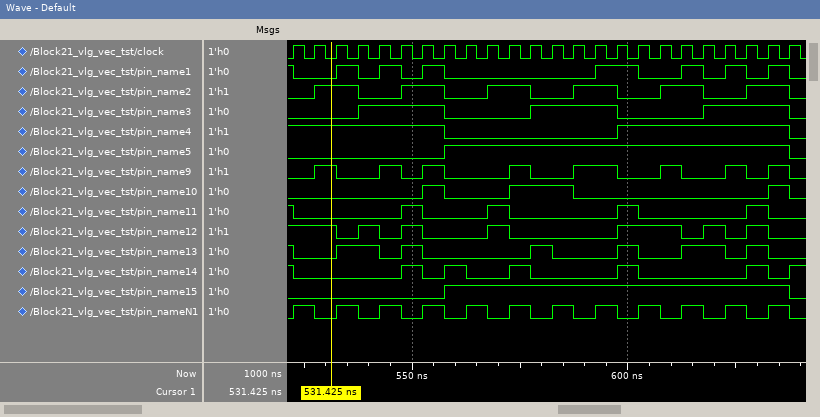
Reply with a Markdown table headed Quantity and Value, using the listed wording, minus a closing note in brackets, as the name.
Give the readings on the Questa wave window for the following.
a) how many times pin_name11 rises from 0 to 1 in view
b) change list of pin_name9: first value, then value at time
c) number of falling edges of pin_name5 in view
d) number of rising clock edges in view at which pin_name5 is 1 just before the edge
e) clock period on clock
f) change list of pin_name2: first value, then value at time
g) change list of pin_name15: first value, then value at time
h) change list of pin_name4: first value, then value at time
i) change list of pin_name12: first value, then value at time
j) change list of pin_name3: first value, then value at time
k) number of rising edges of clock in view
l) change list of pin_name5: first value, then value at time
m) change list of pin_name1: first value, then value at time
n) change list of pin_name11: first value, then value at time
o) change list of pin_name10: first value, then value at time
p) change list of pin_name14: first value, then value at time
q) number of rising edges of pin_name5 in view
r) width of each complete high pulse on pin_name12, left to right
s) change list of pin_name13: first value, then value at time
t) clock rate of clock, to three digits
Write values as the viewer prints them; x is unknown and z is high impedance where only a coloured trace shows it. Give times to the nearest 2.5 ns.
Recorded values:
| Quantity | Value |
|---|---|
| how many times pin_name11 rises from 0 to 1 in view | 4 |
| change list of pin_name9: first value, then value at time | 0, 1 at 527.5 ns, 0 at 532.5 ns, 1 at 542.5 ns, 0 at 547.5 ns, 1 at 552.5 ns, 0 at 557.5 ns, 1 at 572.5 ns, 0 at 577.5 ns, 1 at 587.5 ns, 0 at 597.5 ns, 1 at 607.5 ns, 0 at 612.5 ns, 1 at 622.5 ns, 0 at 627.5 ns, 1 at 632.5 ns, 0 at 637.5 ns |
| number of falling edges of pin_name5 in view | 1 |
| number of rising clock edges in view at which pin_name5 is 1 just before the edge | 16 |
| clock period on clock | 5 ns |
| change list of pin_name2: first value, then value at time | 0, 1 at 527.5 ns, 0 at 537.5 ns, 1 at 547.5 ns, 0 at 557.5 ns, 1 at 567.5 ns, 0 at 577.5 ns, 1 at 587.5 ns, 0 at 597.5 ns, 1 at 607.5 ns, 0 at 617.5 ns, 1 at 627.5 ns, 0 at 637.5 ns |
| change list of pin_name15: first value, then value at time | 0, 1 at 557.5 ns, 0 at 637.5 ns |
| change list of pin_name4: first value, then value at time | 1, 0 at 557.5 ns, 1 at 597.5 ns, 0 at 637.5 ns |
| change list of pin_name12: first value, then value at time | 1, 0 at 532.5 ns, 1 at 537.5 ns, 0 at 542.5 ns, 1 at 547.5 ns, 0 at 552.5 ns, 1 at 567.5 ns, 0 at 572.5 ns, 1 at 597.5 ns, 0 at 612.5 ns, 1 at 617.5 ns, 0 at 622.5 ns, 1 at 627.5 ns, 0 at 632.5 ns |
| change list of pin_name3: first value, then value at time | 0, 1 at 537.5 ns, 0 at 557.5 ns, 1 at 577.5 ns, 0 at 597.5 ns, 1 at 617.5 ns, 0 at 637.5 ns |
| number of rising edges of clock in view | 24 |
| change list of pin_name5: first value, then value at time | 0, 1 at 557.5 ns, 0 at 637.5 ns |
| change list of pin_name1: first value, then value at time | 1, 0 at 522.5 ns, 1 at 532.5 ns, 0 at 537.5 ns, 1 at 542.5 ns, 0 at 547.5 ns, 1 at 552.5 ns, 0 at 557.5 ns, 1 at 592.5 ns, 0 at 602.5 ns, 1 at 612.5 ns, 0 at 617.5 ns, 1 at 622.5 ns, 0 at 627.5 ns, 1 at 632.5 ns, 0 at 637.5 ns |
| change list of pin_name11: first value, then value at time | 1, 0 at 522.5 ns, 1 at 547.5 ns, 0 at 552.5 ns, 1 at 567.5 ns, 0 at 572.5 ns, 1 at 597.5 ns, 0 at 602.5 ns, 1 at 627.5 ns, 0 at 632.5 ns |
| change list of pin_name10: first value, then value at time | 0, 1 at 552.5 ns, 0 at 557.5 ns, 1 at 572.5 ns, 0 at 587.5 ns, 1 at 632.5 ns, 0 at 637.5 ns |
| change list of pin_name14: first value, then value at time | 1, 0 at 522.5 ns, 1 at 547.5 ns, 0 at 552.5 ns, 1 at 557.5 ns, 0 at 562.5 ns, 1 at 572.5 ns, 0 at 577.5 ns, 1 at 597.5 ns, 0 at 602.5 ns, 1 at 627.5 ns, 0 at 632.5 ns, 1 at 637.5 ns |
| number of rising edges of pin_name5 in view | 1 |
| width of each complete high pulse on pin_name12, left to right | 5 ns, 5 ns, 5 ns, 15 ns, 5 ns, 5 ns |
| change list of pin_name13: first value, then value at time | 1, 0 at 522.5 ns, 1 at 532.5 ns, 0 at 542.5 ns, 1 at 547.5 ns, 0 at 552.5 ns, 1 at 577.5 ns, 0 at 582.5 ns, 1 at 597.5 ns, 0 at 602.5 ns, 1 at 612.5 ns, 0 at 622.5 ns, 1 at 627.5 ns, 0 at 632.5 ns |
| clock rate of clock, to three digits | 200 MHz |
